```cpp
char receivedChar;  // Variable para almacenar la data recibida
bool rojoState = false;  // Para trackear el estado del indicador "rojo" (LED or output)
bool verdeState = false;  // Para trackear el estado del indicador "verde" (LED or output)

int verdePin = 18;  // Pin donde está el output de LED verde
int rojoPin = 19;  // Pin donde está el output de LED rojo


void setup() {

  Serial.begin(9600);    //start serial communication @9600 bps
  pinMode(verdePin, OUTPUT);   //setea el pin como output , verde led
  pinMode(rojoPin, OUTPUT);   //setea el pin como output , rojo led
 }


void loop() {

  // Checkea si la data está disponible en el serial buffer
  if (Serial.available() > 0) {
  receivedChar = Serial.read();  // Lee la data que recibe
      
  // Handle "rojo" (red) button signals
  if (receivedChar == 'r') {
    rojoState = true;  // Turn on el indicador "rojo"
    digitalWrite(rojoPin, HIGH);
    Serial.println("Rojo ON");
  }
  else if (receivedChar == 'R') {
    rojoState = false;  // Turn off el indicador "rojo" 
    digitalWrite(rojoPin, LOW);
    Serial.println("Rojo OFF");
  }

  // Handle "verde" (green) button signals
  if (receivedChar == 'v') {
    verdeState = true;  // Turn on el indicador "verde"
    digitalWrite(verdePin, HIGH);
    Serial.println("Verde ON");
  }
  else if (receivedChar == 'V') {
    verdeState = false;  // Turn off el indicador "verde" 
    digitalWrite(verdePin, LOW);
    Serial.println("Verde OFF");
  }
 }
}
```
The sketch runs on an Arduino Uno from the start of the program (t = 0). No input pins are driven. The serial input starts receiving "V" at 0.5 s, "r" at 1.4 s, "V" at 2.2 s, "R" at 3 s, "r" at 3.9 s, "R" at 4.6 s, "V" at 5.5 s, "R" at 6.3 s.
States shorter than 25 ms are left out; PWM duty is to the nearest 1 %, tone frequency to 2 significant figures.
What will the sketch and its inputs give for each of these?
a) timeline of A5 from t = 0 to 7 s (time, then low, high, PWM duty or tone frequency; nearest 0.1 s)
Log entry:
0 s low; 1.4 s high; 3 s low; 3.9 s high; 4.6 s low
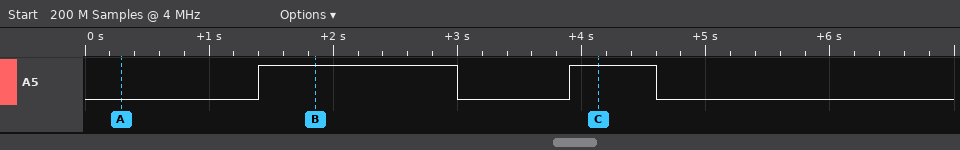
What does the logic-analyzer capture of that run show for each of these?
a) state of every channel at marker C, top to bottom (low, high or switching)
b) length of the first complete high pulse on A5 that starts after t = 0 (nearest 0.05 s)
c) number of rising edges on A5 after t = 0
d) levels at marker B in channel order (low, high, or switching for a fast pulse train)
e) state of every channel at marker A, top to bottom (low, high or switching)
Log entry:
A5 high
1.60 s
2
A5 high
A5 low
